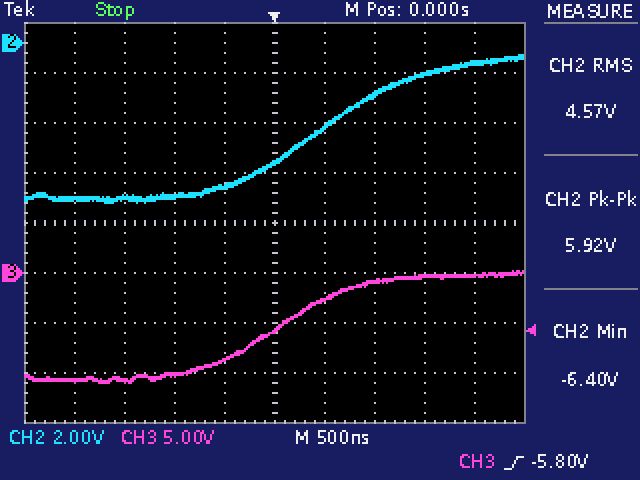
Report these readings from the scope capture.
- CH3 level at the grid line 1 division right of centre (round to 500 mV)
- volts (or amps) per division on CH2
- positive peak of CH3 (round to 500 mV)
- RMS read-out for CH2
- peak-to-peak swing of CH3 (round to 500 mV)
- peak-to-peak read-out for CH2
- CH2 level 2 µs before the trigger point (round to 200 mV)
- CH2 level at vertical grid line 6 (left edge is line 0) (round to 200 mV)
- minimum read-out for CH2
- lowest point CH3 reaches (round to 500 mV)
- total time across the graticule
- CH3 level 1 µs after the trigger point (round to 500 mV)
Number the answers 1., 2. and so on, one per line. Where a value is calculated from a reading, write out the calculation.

1. -2.5 V
2. 2 V
3. 0.0 V
4. 4.57 V
5. 0.0 V − (-11.0 V) = 11.0 V
6. 5.92 V
7. -6.2 V
8. -3.4 V
9. -6.40 V
10. -11.0 V
11. 5 µs
12. -1.0 V
